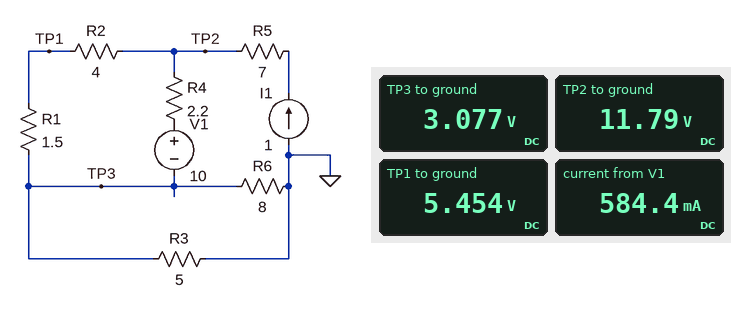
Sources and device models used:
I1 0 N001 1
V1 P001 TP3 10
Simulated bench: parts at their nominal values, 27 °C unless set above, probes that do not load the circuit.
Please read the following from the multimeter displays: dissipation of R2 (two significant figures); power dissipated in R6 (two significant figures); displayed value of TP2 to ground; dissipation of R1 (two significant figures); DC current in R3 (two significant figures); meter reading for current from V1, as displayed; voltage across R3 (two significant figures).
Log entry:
10 W
1.2 W
11.79 V
3.8 W
620 mA
584.4 mA
3.1 V
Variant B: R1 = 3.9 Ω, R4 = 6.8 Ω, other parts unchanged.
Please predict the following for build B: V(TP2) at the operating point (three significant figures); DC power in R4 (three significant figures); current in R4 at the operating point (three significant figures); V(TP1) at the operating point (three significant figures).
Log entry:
12.1 V
139 mW
143 mA
7.53 V
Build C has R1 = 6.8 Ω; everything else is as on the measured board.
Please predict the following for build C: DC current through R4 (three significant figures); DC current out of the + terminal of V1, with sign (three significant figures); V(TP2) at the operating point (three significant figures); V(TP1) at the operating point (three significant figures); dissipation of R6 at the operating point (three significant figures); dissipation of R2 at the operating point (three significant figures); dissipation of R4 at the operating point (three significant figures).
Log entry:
61.5 mA
-61.5 mA
13.2 V
9.46 V
1.18 W
3.52 W
8.33 mW
